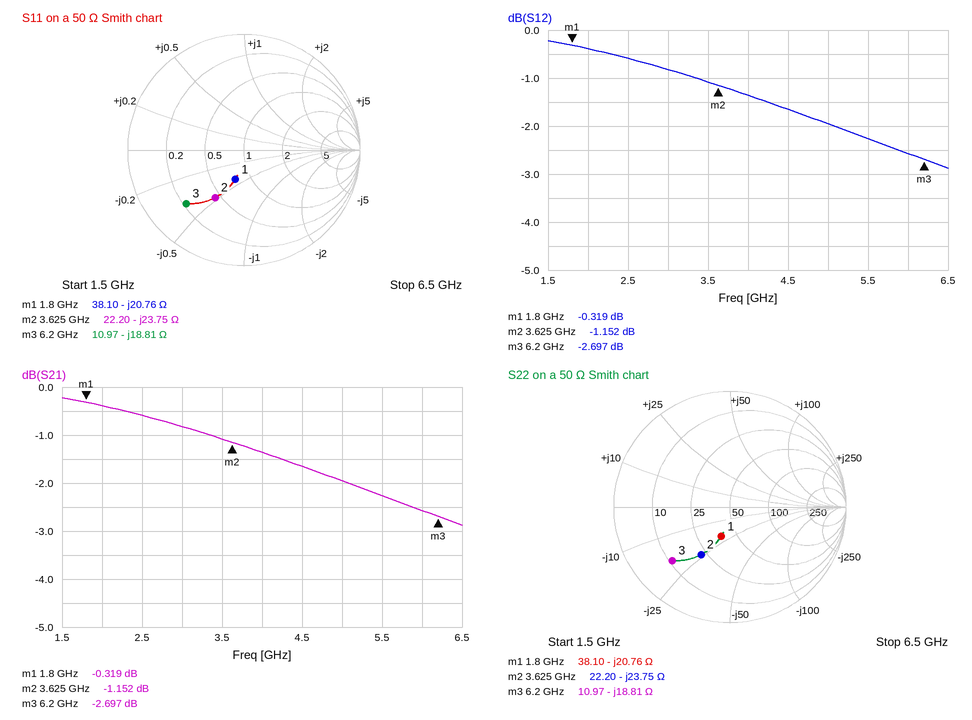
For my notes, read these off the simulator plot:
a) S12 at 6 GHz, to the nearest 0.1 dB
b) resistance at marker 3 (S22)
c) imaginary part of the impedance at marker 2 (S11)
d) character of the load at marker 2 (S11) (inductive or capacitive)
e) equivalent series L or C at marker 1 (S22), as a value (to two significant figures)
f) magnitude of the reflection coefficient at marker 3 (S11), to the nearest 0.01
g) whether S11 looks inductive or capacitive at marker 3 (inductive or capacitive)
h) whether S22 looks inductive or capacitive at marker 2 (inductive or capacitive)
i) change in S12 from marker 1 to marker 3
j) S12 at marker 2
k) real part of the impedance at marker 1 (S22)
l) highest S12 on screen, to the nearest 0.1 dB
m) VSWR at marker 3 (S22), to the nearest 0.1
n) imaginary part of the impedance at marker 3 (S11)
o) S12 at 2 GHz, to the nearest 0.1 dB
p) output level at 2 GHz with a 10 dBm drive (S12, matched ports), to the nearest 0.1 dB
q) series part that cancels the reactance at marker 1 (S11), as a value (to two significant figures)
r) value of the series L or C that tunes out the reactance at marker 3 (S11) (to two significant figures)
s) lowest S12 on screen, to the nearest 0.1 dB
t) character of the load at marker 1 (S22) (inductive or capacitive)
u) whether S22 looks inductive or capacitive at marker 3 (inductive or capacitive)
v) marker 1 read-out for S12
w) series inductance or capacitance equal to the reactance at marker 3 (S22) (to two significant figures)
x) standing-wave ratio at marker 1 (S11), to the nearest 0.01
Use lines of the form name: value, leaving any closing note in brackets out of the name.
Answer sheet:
S12 at 6 GHz, to the nearest 0.1 dB: -2.6 dB
resistance at marker 3: 10.97 Ω
imaginary part of the impedance at marker 2: -23.75 Ω
character of the load at marker 2 (S11): capacitive
equivalent series L or C at marker 1 (S22), as a value: 4.3 pF
magnitude of the reflection coefficient at marker 3 (S11), to the nearest 0.01: 0.68
whether S11 looks inductive or capacitive at marker 3: capacitive
whether S22 looks inductive or capacitive at marker 2: capacitive
change in S12 from marker 1 to marker 3: -2.378 dB
S12 at marker 2: -1.152 dB
real part of the impedance at marker 1: 38.10 Ω
highest S12 on screen, to the nearest 0.1 dB: -0.2 dB
VSWR at marker 3 (S22), to the nearest 0.1: 5.2
imaginary part of the impedance at marker 3: -18.81 Ω
S12 at 2 GHz, to the nearest 0.1 dB: -0.4 dB
output level at 2 GHz with a 10 dBm drive (S12, matched ports), to the nearest 0.1 dB: 9.6 dBm
series part that cancels the reactance at marker 1 (S11), as a value: 1.8 nH
value of the series L or C that tunes out the reactance at marker 3 (S11): 480 pH
lowest S12 on screen, to the nearest 0.1 dB: -2.9 dB
character of the load at marker 1 (S22): capacitive
whether S22 looks inductive or capacitive at marker 3: capacitive
marker 1 read-out for S12: -0.319 dB
series inductance or capacitance equal to the reactance at marker 3 (S22): 1.4 pF
standing-wave ratio at marker 1 (S11), to the nearest 0.01: 1.72
